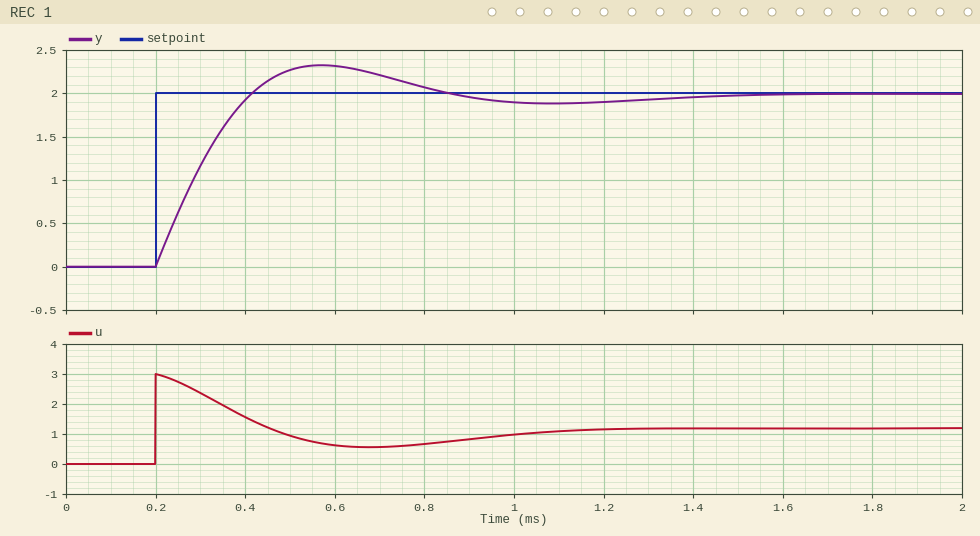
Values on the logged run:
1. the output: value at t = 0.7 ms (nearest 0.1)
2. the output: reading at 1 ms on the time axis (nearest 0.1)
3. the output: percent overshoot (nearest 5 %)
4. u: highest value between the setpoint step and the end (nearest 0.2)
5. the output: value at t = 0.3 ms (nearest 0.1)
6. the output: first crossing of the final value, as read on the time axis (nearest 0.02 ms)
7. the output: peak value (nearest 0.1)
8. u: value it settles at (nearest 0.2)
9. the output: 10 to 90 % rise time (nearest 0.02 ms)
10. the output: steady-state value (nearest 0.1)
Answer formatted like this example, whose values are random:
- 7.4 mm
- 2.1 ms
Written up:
- 2.2
- 1.9
- 15 %
- 3.0
- 1.2
- 0.42 ms
- 2.3
- 1.2
- 0.16 ms
- 2.0
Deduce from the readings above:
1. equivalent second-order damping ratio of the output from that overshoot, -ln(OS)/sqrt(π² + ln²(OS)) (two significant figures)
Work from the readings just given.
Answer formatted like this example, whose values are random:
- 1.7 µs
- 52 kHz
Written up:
- 0.52
